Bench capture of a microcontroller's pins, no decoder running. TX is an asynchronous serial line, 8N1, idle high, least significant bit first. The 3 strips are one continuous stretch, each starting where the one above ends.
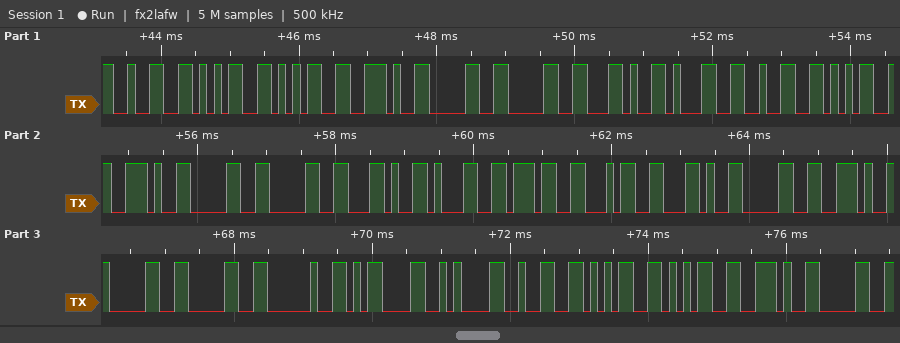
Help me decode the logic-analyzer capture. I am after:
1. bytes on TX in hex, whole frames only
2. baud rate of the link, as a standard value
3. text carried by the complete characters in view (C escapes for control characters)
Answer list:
0x32 0x35 0x35 0x2E 0x30 0x30 0x2C 0x31 0x32 0x35 0x2E 0x30 0x30 0x2C 0x31 0x37 0x34 0x2C 0x30 0x2E 0x30 0x30 0x20 0x0D 0x0A 0x32 0x35 0x35 0x2E 0x30
9600 baud
"255.00,125.00,174,0.00 \r\n255.0"
